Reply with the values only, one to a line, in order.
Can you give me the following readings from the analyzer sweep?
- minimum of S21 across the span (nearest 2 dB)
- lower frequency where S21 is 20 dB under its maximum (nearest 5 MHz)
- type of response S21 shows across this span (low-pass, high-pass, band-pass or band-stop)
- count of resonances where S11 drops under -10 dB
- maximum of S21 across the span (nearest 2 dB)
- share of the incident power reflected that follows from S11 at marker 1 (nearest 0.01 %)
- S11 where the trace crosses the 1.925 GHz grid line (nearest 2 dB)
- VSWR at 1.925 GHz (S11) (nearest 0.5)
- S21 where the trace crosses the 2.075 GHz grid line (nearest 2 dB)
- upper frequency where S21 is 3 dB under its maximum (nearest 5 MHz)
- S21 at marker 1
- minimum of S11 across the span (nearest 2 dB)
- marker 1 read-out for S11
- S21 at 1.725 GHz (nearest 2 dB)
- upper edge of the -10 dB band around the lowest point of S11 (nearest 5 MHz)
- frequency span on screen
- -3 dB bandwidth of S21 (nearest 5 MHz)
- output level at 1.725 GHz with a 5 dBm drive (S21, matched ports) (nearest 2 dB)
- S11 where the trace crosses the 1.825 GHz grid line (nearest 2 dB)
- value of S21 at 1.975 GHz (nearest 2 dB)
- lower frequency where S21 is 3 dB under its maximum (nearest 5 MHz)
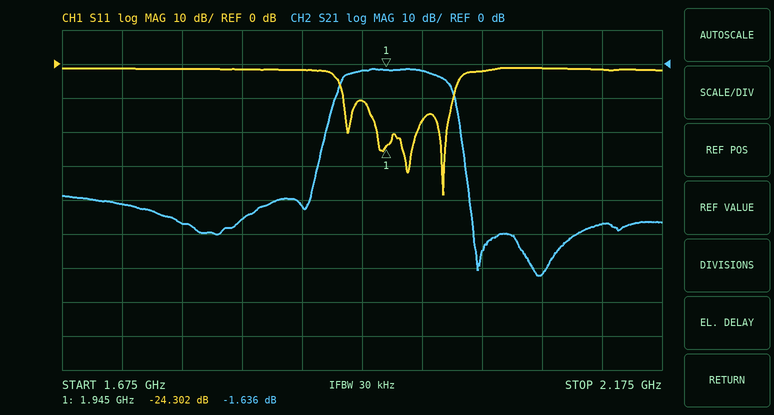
-62 dB
1.895 GHz
band-pass
4
-2 dB
0.37 %
-10 dB
2.0
-62 dB
1.995 GHz
-1.636 dB
-38 dB
-24.302 dB
-42 dB
2.000 GHz
500 MHz
85 MHz
-36 dBm
-2 dB
-2 dB
1.910 GHz
